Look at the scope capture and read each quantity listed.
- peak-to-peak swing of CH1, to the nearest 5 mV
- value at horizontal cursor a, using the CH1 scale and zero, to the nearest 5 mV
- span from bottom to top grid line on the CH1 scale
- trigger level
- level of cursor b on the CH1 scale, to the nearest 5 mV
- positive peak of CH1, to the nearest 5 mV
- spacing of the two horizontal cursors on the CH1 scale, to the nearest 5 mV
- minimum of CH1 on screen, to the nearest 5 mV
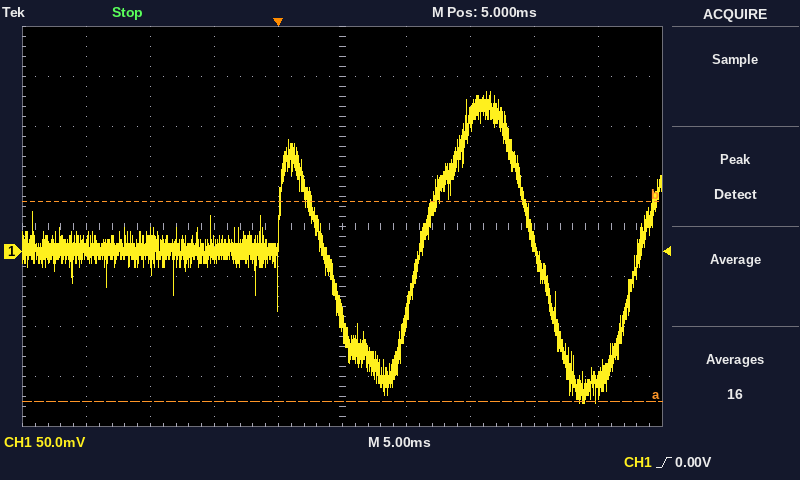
310 mV
-150 mV
400 mV
0.00 V
50 mV
160 mV
200 mV
-150 mV
